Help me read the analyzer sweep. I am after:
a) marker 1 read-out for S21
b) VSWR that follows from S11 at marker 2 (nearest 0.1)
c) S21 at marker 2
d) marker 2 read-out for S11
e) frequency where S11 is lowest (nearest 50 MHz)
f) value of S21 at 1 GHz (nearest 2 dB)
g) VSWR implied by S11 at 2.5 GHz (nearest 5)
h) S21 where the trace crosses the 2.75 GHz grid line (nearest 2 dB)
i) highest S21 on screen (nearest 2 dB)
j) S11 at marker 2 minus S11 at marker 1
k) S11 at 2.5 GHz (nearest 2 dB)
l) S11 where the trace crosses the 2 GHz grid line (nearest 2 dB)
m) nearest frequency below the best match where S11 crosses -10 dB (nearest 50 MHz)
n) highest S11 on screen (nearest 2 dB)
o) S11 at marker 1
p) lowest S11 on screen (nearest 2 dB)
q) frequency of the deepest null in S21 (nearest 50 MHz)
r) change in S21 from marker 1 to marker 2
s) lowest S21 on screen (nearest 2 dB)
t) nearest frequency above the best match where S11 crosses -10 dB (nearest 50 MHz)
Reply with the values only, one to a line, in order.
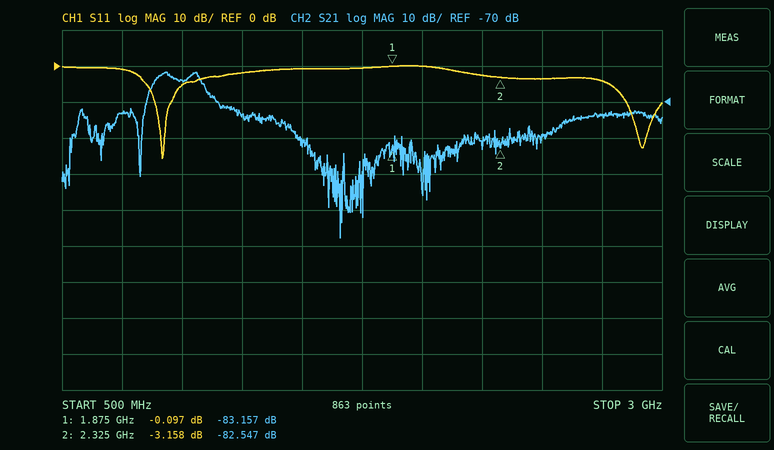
-83.157 dB
5.6
-82.547 dB
-3.158 dB
900 MHz
-64 dB
5
-74 dB
-62 dB
-3.061 dB
-4 dB
0 dB
900 MHz
0 dB
-0.097 dB
-26 dB
1.65 GHz
0.610 dB
-108 dB
950 MHz
